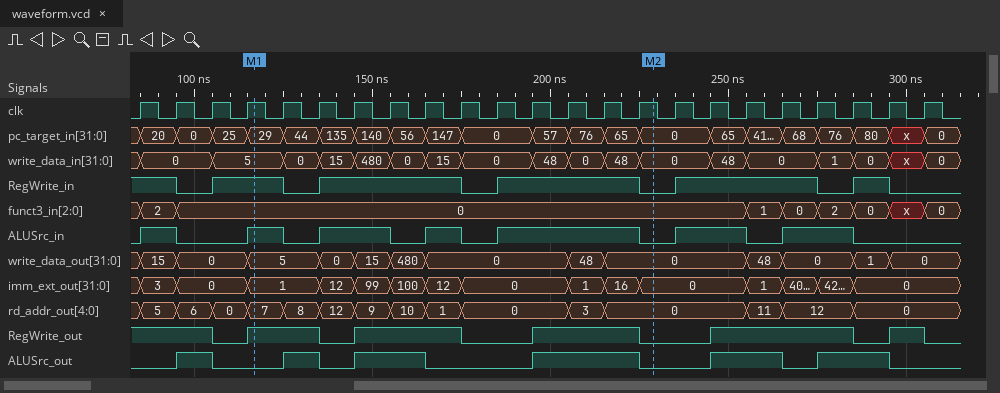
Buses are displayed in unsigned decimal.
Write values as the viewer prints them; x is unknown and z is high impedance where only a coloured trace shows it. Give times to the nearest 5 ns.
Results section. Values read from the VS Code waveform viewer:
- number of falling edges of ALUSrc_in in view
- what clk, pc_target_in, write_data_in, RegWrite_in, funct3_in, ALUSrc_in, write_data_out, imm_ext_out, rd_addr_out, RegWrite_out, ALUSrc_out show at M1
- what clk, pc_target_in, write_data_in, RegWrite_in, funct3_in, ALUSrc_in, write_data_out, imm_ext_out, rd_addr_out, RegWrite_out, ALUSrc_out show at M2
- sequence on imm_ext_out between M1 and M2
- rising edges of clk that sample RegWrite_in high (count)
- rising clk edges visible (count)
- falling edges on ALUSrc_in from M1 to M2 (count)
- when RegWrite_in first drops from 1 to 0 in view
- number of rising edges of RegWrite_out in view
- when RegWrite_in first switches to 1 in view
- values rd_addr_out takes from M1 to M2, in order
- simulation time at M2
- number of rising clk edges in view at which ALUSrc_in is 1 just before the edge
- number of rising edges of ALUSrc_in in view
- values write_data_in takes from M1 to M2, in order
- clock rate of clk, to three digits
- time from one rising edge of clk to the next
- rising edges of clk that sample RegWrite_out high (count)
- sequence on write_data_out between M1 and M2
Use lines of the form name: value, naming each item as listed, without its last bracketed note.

number of falling edges of ALUSrc_in in view: 7
what clk, pc_target_in, write_data_in, RegWrite_in, funct3_in, ALUSrc_in, write_data_out, imm_ext_out, rd_addr_out, RegWrite_out, ALUSrc_out show at M1: clk=1, pc_target_in=29, write_data_in=5, RegWrite_in=1, funct3_in=0, ALUSrc_in=1, write_data_out=5, imm_ext_out=1, rd_addr_out=7, RegWrite_out=1, ALUSrc_out=0
what clk, pc_target_in, write_data_in, RegWrite_in, funct3_in, ALUSrc_in, write_data_out, imm_ext_out, rd_addr_out, RegWrite_out, ALUSrc_out show at M2: clk=1, pc_target_in=0, write_data_in=0, RegWrite_in=0, funct3_in=0, ALUSrc_in=0, write_data_out=0, imm_ext_out=0, rd_addr_out=0, RegWrite_out=0, ALUSrc_out=0
sequence on imm_ext_out between M1 and M2: 1, 12, 99, 100, 12, 0, 1, 16, 0
rising edges of clk that sample RegWrite_in high: 17
rising clk edges visible: 23
falling edges on ALUSrc_in from M1 to M2: 4
when RegWrite_in first drops from 1 to 0 in view: 95 ns
number of rising edges of RegWrite_out in view: 5
when RegWrite_in first switches to 1 in view: 105 ns
values rd_addr_out takes from M1 to M2, in order: 7, 8, 12, 9, 10, 1, 0, 3, 0
simulation time at M2: 230 ns
number of rising clk edges in view at which ALUSrc_in is 1 just before the edge: 13
number of rising edges of ALUSrc_in in view: 7
values write_data_in takes from M1 to M2, in order: 5, 0, 15, 480, 0, 15, 0, 48, 0, 48, 0
clock rate of clk, to three digits: 100 MHz
time from one rising edge of clk to the next: 10 ns
rising edges of clk that sample RegWrite_out high: 16
sequence on write_data_out between M1 and M2: 5, 0, 15, 480, 0, 48, 0
